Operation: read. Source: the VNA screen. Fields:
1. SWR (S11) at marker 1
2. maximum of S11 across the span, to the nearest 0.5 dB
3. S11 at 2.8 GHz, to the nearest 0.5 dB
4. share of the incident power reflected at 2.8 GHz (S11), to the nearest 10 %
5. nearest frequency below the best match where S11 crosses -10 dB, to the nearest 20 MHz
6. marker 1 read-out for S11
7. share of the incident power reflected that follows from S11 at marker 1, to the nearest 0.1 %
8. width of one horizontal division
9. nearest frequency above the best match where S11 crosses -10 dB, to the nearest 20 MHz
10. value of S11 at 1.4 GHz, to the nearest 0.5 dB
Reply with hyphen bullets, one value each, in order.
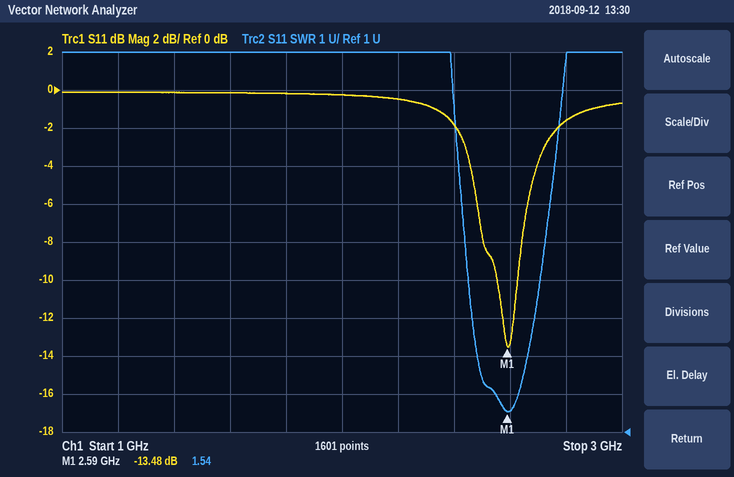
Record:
- 1.54
- 0.0 dB
- -1.5 dB
- 70 %
- 2.56 GHz
- -13.48 dB
- 4.5 %
- 200 MHz
- 2.62 GHz
- 0.0 dB
